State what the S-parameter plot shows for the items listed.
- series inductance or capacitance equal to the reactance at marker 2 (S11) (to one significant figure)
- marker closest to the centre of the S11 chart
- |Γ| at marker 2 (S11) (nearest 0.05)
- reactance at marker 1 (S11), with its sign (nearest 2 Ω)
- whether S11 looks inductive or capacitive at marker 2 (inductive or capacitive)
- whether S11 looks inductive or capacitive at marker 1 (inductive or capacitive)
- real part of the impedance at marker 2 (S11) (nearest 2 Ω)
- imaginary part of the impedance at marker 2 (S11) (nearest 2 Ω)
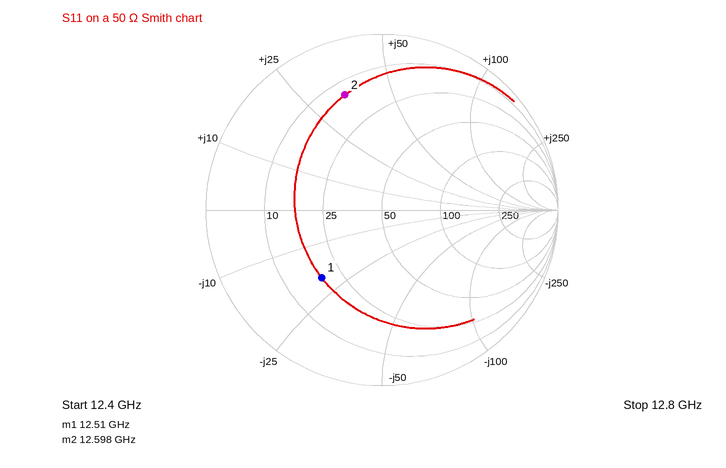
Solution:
400 pH
marker 1
0.70
-20 Ω
inductive
capacitive
14 Ω
+34 Ω
